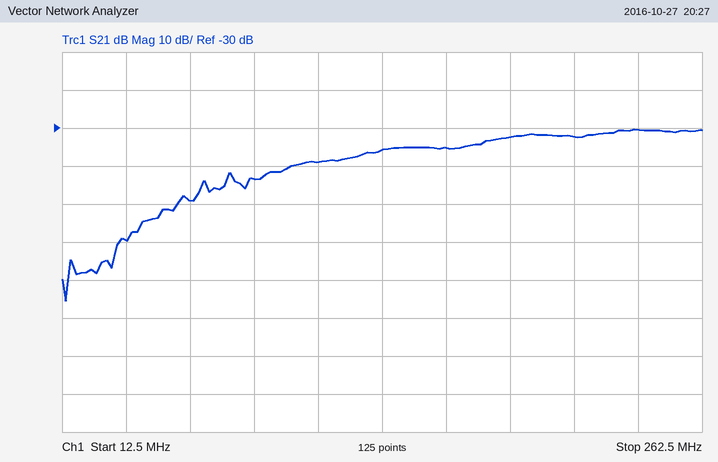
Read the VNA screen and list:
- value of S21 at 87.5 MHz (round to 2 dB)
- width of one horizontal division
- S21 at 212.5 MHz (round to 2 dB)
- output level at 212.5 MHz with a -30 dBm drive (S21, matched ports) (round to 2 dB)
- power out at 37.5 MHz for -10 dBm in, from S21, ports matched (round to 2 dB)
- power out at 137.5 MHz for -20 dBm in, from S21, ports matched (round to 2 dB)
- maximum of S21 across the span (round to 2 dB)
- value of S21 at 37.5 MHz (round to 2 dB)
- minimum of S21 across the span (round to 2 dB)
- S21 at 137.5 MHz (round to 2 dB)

-44 dB
25 MHz
-32 dB
-62 dBm
-70 dBm
-56 dBm
-30 dB
-60 dB
-76 dB
-36 dB
